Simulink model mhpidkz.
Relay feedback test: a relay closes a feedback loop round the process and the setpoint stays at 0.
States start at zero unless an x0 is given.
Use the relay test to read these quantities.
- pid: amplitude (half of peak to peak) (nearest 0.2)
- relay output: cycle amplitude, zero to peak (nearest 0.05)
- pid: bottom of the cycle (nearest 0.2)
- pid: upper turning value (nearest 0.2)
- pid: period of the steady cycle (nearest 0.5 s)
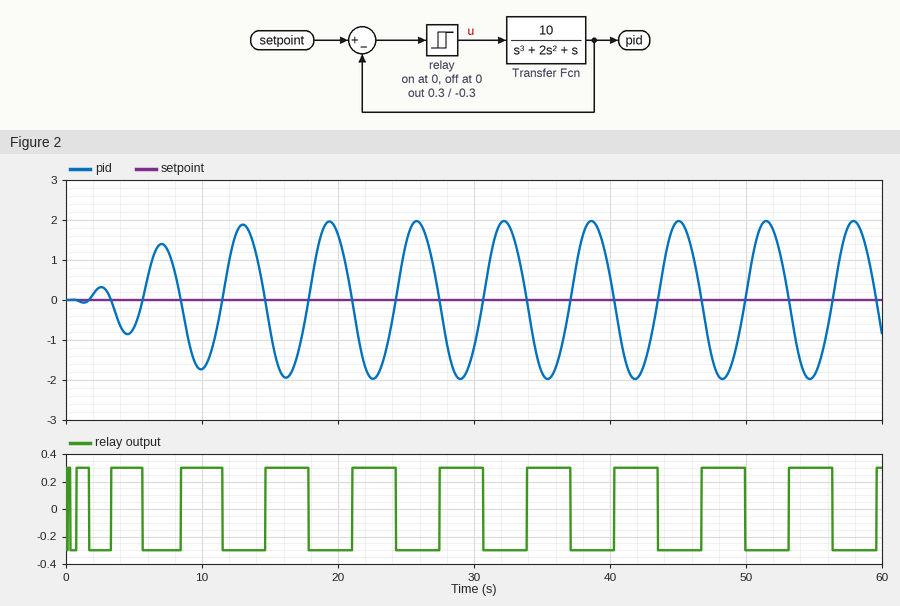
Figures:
2.0
0.30
-2.0
2.0
6.5 s
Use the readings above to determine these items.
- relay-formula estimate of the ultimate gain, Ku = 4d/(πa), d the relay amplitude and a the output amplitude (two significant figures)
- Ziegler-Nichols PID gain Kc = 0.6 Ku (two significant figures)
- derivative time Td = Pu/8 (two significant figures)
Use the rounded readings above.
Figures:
0.19
0.11
0.81 s
